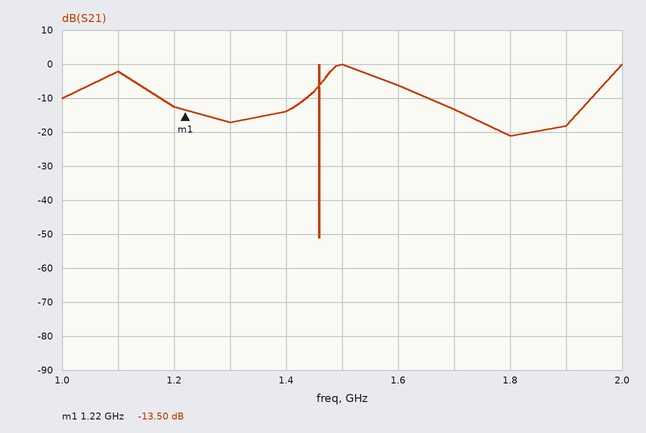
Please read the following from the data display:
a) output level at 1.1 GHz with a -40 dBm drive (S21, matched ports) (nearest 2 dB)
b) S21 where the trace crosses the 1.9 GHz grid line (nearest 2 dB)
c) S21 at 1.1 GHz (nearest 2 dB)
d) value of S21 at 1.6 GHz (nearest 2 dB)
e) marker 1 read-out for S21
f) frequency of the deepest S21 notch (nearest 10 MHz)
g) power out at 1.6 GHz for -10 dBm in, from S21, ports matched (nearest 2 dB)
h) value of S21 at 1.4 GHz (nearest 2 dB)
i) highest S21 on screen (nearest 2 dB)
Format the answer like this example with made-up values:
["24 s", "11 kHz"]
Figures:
["-42 dBm", "-18 dB", "-2 dB", "-6 dB", "-13.50 dB", "1.46 GHz", "-16 dBm", "-14 dB", "0 dB"]
